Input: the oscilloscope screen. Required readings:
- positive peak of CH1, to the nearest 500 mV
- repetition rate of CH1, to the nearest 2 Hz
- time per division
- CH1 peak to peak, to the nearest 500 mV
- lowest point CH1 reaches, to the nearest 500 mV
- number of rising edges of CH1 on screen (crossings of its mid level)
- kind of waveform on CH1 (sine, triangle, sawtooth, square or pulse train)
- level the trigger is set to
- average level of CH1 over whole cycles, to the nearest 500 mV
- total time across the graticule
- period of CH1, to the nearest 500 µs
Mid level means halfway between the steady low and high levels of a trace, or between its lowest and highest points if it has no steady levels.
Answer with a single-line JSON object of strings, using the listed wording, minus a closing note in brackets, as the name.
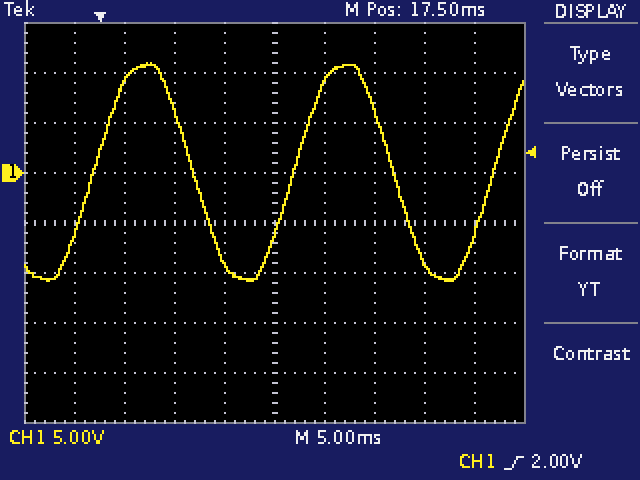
{"positive peak of CH1, to the nearest 500 mV": "11.0 V", "repetition rate of CH1, to the nearest 2 Hz": "50 Hz", "time per division": "5 ms", "CH1 peak to peak, to the nearest 500 mV": "22.0 V", "lowest point CH1 reaches, to the nearest 500 mV": "-11.0 V", "number of rising edges of CH1 on screen": "3", "kind of waveform on CH1": "sine", "level the trigger is set to": "2.00 V", "average level of CH1 over whole cycles, to the nearest 500 mV": "0.0 V", "total time across the graticule": "50 ms", "period of CH1, to the nearest 500 µs": "20.0 ms"}
